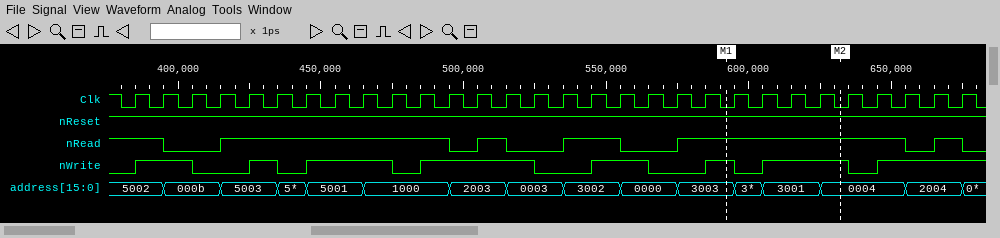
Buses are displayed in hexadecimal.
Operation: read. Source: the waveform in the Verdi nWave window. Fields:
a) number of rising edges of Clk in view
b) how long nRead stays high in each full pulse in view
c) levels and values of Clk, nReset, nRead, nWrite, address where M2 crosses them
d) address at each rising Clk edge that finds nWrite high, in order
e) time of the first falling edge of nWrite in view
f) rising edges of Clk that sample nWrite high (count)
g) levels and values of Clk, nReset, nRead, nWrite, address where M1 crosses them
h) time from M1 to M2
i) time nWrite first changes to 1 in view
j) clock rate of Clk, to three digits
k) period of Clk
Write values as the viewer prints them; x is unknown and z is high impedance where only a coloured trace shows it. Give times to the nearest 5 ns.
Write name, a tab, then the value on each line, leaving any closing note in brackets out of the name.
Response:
number of rising edges of Clk in view	30
how long nRead stays high in each full pulse in view	80 ns, 10 ns, 20 ns, 80 ns, 10 ns
levels and values of Clk, nReset, nRead, nWrite, address where M2 crosses them	Clk=0, nReset=1, nRead=1, nWrite=1, address=0004
address at each rising Clk edge that finds nWrite high, in order	5002, 000b, 5003, 5001, 5001, 1000, 1000, 2003, 2003, 0003, 3002, 0000, 3003, 3001, 3001, 0004, 0004, 2004, 2004
time of the first falling edge of nWrite in view	405 ns
rising edges of Clk that sample nWrite high	19
levels and values of Clk, nReset, nRead, nWrite, address where M1 crosses them	Clk=0, nReset=1, nRead=1, nWrite=1, address=3003
time from M1 to M2	40 ns
time nWrite first changes to 1 in view	385 ns
clock rate of Clk, to three digits	100 MHz
period of Clk	10 ns
